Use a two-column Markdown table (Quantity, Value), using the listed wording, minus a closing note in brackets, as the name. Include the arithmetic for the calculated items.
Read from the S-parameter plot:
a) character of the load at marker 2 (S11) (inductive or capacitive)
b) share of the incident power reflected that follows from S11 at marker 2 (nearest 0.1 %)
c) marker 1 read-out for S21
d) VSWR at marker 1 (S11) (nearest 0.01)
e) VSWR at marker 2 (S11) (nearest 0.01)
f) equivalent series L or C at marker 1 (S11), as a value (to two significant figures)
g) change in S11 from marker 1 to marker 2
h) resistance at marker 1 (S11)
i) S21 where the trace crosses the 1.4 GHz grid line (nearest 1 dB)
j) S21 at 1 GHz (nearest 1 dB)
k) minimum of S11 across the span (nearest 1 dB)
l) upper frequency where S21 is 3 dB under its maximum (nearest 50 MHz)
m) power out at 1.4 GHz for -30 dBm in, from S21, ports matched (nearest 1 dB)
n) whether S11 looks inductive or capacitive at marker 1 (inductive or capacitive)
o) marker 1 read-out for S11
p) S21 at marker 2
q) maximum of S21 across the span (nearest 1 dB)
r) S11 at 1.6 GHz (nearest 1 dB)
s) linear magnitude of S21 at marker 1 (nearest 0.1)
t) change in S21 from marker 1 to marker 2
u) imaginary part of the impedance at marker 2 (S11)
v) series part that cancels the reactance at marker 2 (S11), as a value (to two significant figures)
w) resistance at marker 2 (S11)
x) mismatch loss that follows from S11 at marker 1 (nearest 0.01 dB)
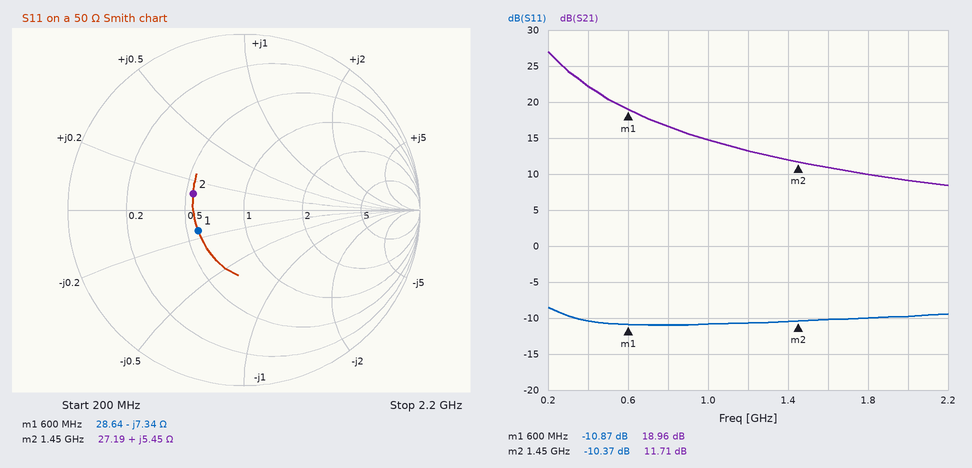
| Quantity | Value |
|---|---|
| character of the load at marker 2 (S11) | inductive |
| share of the incident power reflected that follows from S11 at marker 2 | 10^(-10.37/10) ≈ 9.2 % |
| marker 1 read-out for S21 | 18.96 dB |
| VSWR at marker 1 (S11) | 1.80 |
| VSWR at marker 2 (S11) | 1.87 |
| equivalent series L or C at marker 1 (S11), as a value | C = 1/(2π × 600 MHz × 7.34 Ω) ≈ 36 pF |
| change in S11 from marker 1 to marker 2 | -10.37 − (-10.87) = 0.50 dB |
| resistance at marker 1 | 28.64 Ω |
| S21 where the trace crosses the 1.4 GHz grid line | 12 dB |
| S21 at 1 GHz | 15 dB |
| minimum of S11 across the span | -11 dB |
| upper frequency where S21 is 3 dB under its maximum | 300 MHz |
| power out at 1.4 GHz for -30 dBm in, from S21, ports matched | -30 dBm + (12 dB) = -18 dBm |
| whether S11 looks inductive or capacitive at marker 1 | capacitive |
| marker 1 read-out for S11 | -10.87 dB |
| S21 at marker 2 | 11.71 dB |
| maximum of S21 across the span | 27 dB |
| S11 at 1.6 GHz | -10 dB |
| linear magnitude of S21 at marker 1 | 10^(18.96/20) ≈ 8.9 |
| change in S21 from marker 1 to marker 2 | 11.71 − (18.96) = -7.25 dB |
| imaginary part of the impedance at marker 2 | +5.45 Ω |
| series part that cancels the reactance at marker 2 (S11), as a value | C = 1/(2π × 1.45 GHz × 5.45 Ω) ≈ 20 pF |
| resistance at marker 2 | 27.19 Ω |
| mismatch loss that follows from S11 at marker 1 | −10 log10(1 − 10^(-10.87/10)) ≈ 0.37 dB |
